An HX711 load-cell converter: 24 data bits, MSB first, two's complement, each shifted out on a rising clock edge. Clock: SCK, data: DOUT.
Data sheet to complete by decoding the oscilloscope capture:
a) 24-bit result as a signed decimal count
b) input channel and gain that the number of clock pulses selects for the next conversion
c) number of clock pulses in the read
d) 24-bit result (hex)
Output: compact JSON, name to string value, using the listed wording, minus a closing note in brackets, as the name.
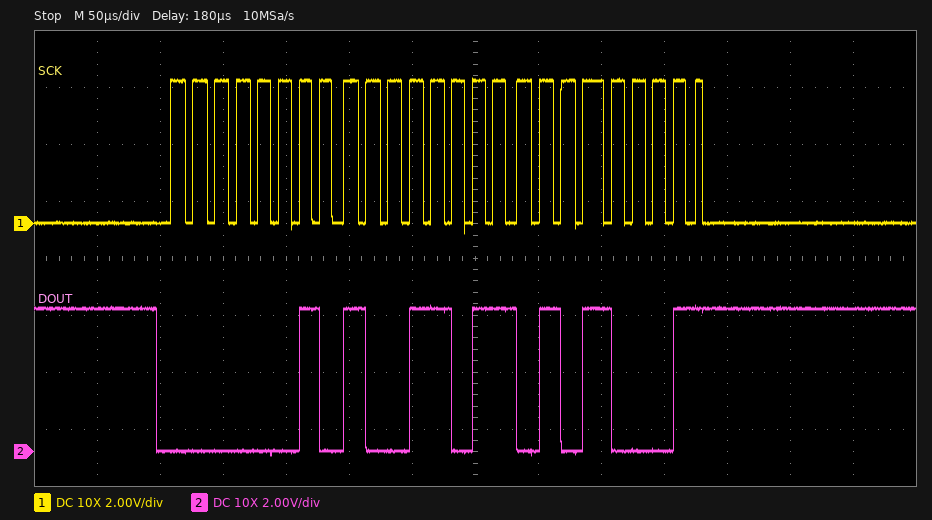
{"24-bit result as a signed decimal count": "170833", "input channel and gain that the number of clock pulses selects for the next conversion": "channel A, gain 128", "number of clock pulses in the read": "25", "24-bit result": "0x029B51"}
